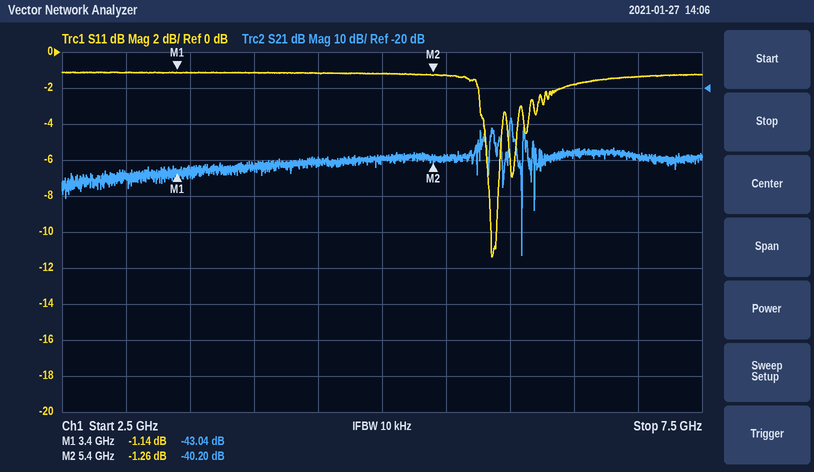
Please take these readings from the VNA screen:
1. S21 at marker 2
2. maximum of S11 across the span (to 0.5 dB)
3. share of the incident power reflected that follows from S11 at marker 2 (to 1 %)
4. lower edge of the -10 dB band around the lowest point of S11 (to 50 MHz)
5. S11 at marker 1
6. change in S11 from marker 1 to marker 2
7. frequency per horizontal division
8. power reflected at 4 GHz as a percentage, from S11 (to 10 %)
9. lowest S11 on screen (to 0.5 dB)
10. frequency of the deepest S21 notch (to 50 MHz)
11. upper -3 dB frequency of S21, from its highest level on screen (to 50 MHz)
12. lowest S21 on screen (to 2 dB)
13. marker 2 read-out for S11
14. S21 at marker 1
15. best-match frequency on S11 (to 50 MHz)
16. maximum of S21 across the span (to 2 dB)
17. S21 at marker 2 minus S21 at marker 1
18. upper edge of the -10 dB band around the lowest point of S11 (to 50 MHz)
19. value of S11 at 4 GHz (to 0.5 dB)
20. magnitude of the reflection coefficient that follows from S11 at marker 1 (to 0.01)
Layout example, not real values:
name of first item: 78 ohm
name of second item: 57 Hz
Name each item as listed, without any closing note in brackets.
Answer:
S21 at marker 2: -40.20 dB
maximum of S11 across the span: -1.0 dB
share of the incident power reflected that follows from S11 at marker 2: 75 %
lower edge of the -10 dB band around the lowest point of S11: 5.85 GHz
S11 at marker 1: -1.14 dB
change in S11 from marker 1 to marker 2: -0.12 dB
frequency per horizontal division: 500 MHz
power reflected at 4 GHz as a percentage, from S11: 80 %
lowest S11 on screen: -11.5 dB
frequency of the deepest S21 notch: 6.10 GHz
upper -3 dB frequency of S21, from its highest level on screen: 6.00 GHz
lowest S21 on screen: -66 dB
marker 2 read-out for S11: -1.26 dB
S21 at marker 1: -43.04 dB
best-match frequency on S11: 5.85 GHz
maximum of S21 across the span: -28 dB
S21 at marker 2 minus S21 at marker 1: 2.84 dB
upper edge of the -10 dB band around the lowest point of S11: 5.90 GHz
value of S11 at 4 GHz: -1.0 dB
magnitude of the reflection coefficient that follows from S11 at marker 1: 0.88
